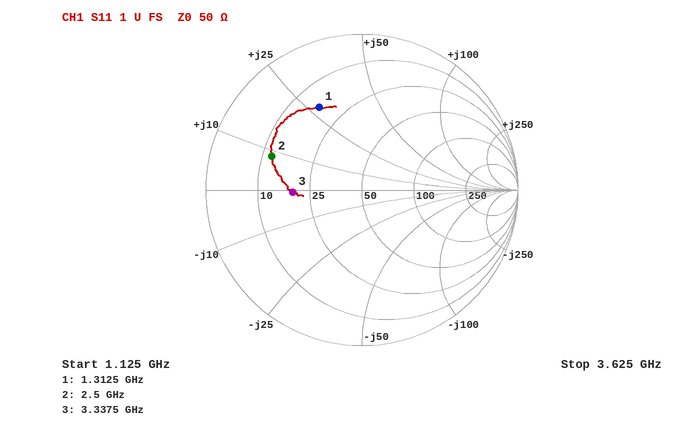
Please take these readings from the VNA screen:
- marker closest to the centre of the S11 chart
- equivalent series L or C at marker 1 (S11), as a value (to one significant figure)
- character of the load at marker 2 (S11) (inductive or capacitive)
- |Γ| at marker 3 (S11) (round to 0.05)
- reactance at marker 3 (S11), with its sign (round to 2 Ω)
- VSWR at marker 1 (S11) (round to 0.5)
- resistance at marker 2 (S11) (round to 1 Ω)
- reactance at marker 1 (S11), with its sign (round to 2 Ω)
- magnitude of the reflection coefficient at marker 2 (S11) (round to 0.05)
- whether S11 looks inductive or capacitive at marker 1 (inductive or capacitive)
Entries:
marker 3
3 nH
inductive
0.45
0 Ω
4.0
12 Ω
+28 Ω
0.60
inductive
